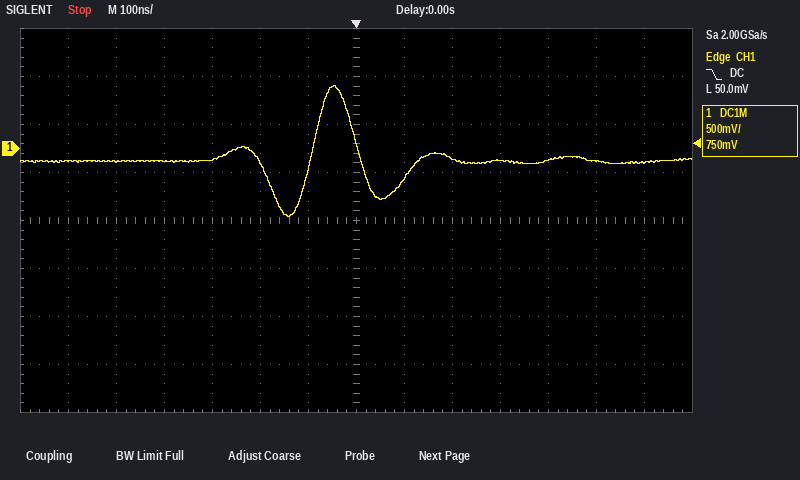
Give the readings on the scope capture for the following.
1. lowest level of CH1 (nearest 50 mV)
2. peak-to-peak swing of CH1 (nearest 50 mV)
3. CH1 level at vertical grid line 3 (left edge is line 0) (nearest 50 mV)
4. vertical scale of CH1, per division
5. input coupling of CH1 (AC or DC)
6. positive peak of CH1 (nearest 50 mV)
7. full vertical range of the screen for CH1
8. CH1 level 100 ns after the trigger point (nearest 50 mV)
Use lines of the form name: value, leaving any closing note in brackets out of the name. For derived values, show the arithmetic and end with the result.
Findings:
lowest level of CH1: -700 mV
peak-to-peak swing of CH1: 650 mV − (-700 mV) = 1.35 V
CH1 level at vertical grid line 3 (left edge is line 0): -150 mV
vertical scale of CH1, per division: 500 mV
input coupling of CH1: DC
positive peak of CH1: 650 mV
full vertical range of the screen for CH1: 4 V
CH1 level 100 ns after the trigger point: -300 mV
